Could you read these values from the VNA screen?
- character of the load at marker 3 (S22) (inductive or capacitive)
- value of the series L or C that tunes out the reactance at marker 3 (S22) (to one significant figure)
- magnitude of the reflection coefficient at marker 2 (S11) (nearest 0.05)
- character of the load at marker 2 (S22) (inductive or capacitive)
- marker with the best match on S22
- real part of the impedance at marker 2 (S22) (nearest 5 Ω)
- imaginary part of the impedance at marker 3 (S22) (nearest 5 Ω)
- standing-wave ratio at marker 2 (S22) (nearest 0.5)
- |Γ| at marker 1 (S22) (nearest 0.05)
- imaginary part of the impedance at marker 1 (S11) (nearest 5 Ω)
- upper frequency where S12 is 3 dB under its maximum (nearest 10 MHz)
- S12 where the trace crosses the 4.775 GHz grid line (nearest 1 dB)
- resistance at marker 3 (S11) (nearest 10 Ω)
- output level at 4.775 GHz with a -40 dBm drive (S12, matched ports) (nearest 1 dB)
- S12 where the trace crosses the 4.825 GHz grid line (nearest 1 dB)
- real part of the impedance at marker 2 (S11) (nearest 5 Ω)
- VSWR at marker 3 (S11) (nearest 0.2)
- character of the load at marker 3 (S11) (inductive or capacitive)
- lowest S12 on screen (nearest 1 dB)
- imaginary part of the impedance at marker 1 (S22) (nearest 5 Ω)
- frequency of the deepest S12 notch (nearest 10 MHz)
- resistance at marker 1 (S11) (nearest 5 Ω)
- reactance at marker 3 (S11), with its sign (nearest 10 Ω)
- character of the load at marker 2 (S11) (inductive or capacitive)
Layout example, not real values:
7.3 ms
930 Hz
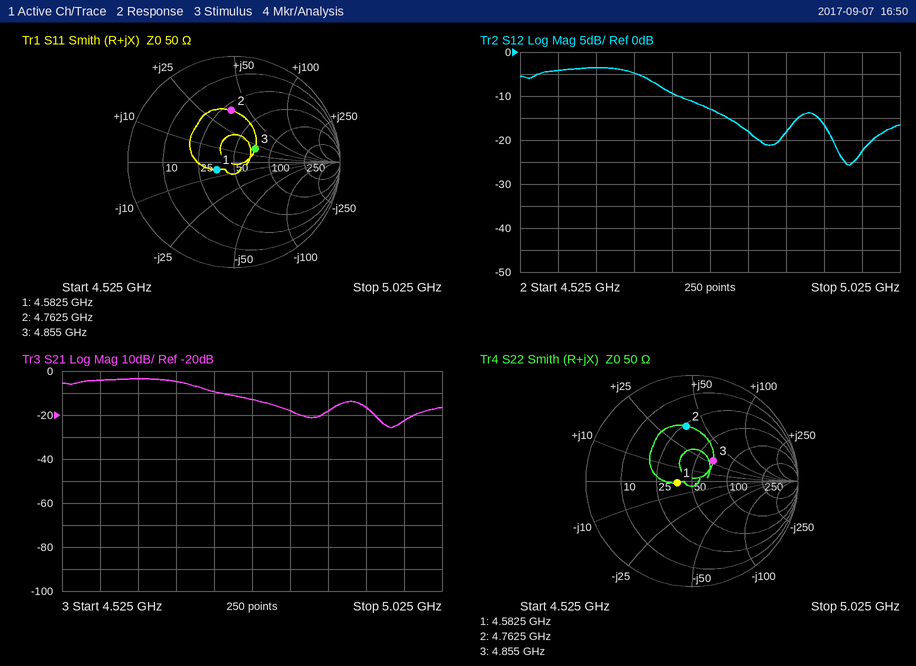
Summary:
inductive
1 pF
0.50
inductive
marker 1
25 Ω
+30 Ω
3.0
0.15
-5 Ω
4.70 GHz
-13 dB
70 Ω
-53 dBm
-18 dB
30 Ω
1.6
inductive
-26 dB
0 Ω
4.96 GHz
35 Ω
+20 Ω
inductive
